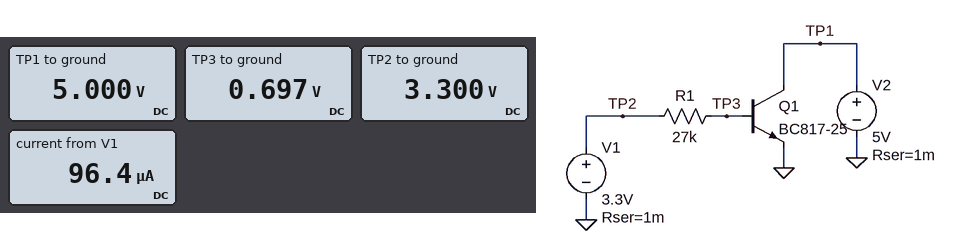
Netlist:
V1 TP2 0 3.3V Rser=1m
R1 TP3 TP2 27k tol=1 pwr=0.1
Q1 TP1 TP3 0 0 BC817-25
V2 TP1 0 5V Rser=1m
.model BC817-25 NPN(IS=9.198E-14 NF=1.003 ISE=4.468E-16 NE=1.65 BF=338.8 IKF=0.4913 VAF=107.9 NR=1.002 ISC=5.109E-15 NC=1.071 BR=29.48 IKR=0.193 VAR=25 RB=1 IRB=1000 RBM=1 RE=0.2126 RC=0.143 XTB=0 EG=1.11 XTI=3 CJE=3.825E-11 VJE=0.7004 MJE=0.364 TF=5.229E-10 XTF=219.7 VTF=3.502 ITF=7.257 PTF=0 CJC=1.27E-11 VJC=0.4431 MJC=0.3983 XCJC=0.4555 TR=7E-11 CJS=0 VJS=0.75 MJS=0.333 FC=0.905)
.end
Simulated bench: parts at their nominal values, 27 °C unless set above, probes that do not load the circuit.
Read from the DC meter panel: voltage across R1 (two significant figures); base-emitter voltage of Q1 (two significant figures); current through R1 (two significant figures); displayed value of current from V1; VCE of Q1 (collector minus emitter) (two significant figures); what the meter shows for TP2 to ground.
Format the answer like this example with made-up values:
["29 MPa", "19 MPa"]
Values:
["2.6 V", "700 mV", "96 µA", "96.4 µA", "5.0 V", "3.300 V"]
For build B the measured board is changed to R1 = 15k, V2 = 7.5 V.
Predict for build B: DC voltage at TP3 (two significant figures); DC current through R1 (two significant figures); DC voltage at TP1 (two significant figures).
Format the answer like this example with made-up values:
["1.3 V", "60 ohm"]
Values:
["720 mV", "170 µA", "7.5 V"]
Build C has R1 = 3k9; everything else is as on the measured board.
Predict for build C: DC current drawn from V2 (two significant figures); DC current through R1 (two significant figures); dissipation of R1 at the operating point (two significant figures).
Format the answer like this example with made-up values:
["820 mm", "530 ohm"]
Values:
["170 mA", "650 µA", "1.6 mW"]
